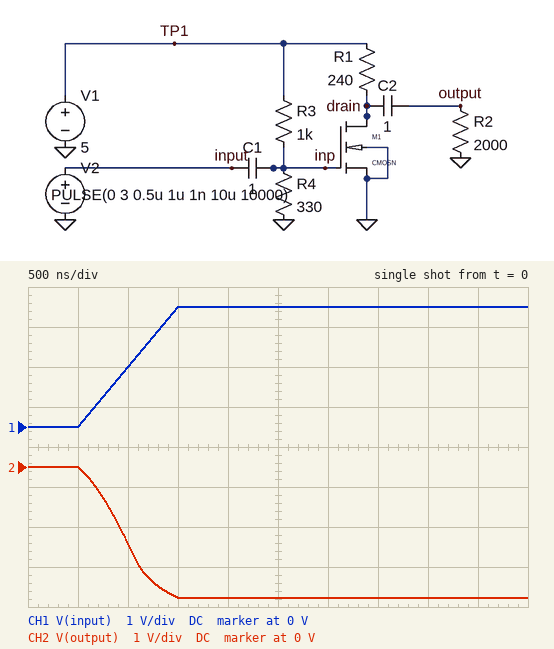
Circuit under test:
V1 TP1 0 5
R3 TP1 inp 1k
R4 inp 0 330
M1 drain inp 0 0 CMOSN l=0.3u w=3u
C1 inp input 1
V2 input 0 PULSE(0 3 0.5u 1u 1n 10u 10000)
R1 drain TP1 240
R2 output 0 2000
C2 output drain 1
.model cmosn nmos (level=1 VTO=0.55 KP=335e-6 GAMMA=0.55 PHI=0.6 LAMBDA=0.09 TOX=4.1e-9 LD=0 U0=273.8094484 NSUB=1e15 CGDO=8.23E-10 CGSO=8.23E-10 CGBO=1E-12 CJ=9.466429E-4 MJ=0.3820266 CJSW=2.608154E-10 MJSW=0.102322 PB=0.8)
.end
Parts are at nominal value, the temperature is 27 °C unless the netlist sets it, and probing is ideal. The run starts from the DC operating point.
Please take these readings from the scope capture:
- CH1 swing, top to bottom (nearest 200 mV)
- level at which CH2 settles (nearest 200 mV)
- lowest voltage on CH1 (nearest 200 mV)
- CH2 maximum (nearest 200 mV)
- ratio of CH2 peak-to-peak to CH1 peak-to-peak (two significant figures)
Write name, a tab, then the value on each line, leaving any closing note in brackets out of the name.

CH1 swing, top to bottom	3.0 V
level at which CH2 settles	-3.2 V
lowest voltage on CH1	0 V
CH2 maximum	0 V
ratio of CH2 peak-to-peak to CH1 peak-to-peak	1.1
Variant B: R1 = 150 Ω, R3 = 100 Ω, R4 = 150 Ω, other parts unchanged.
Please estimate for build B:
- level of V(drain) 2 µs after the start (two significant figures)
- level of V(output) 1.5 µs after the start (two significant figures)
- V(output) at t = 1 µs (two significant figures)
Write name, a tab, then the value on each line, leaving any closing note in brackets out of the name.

level of V(drain) 2 µs after the start	1.4 V
level of V(output) 1.5 µs after the start	-1.7 V
V(output) at t = 1 µs	-1.2 V
